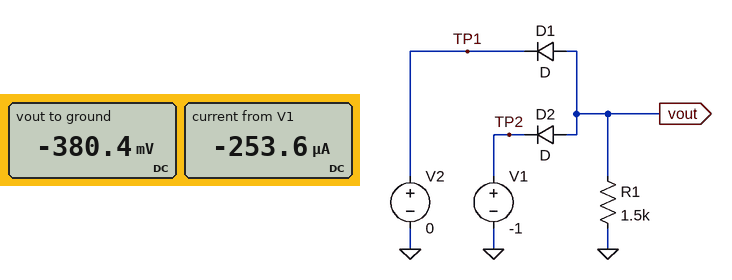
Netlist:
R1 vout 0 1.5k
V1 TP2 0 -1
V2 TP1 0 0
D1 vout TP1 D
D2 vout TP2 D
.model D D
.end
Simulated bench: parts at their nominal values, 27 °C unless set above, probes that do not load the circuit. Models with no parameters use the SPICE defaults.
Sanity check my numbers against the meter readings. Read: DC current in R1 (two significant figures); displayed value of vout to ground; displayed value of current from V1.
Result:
250 µA
-380.4 mV
-253.6 µA
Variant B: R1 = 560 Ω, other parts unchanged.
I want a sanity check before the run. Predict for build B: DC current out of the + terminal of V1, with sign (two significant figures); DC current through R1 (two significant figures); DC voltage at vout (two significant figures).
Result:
-640 µA
640 µA
-360 mV
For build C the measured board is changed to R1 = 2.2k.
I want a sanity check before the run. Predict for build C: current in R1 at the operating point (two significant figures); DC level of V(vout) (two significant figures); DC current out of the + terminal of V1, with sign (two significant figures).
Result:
180 µA
-390 mV
-180 µA
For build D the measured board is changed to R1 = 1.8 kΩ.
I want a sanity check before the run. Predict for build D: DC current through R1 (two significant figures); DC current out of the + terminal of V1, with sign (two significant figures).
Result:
210 µA
-210 µA
